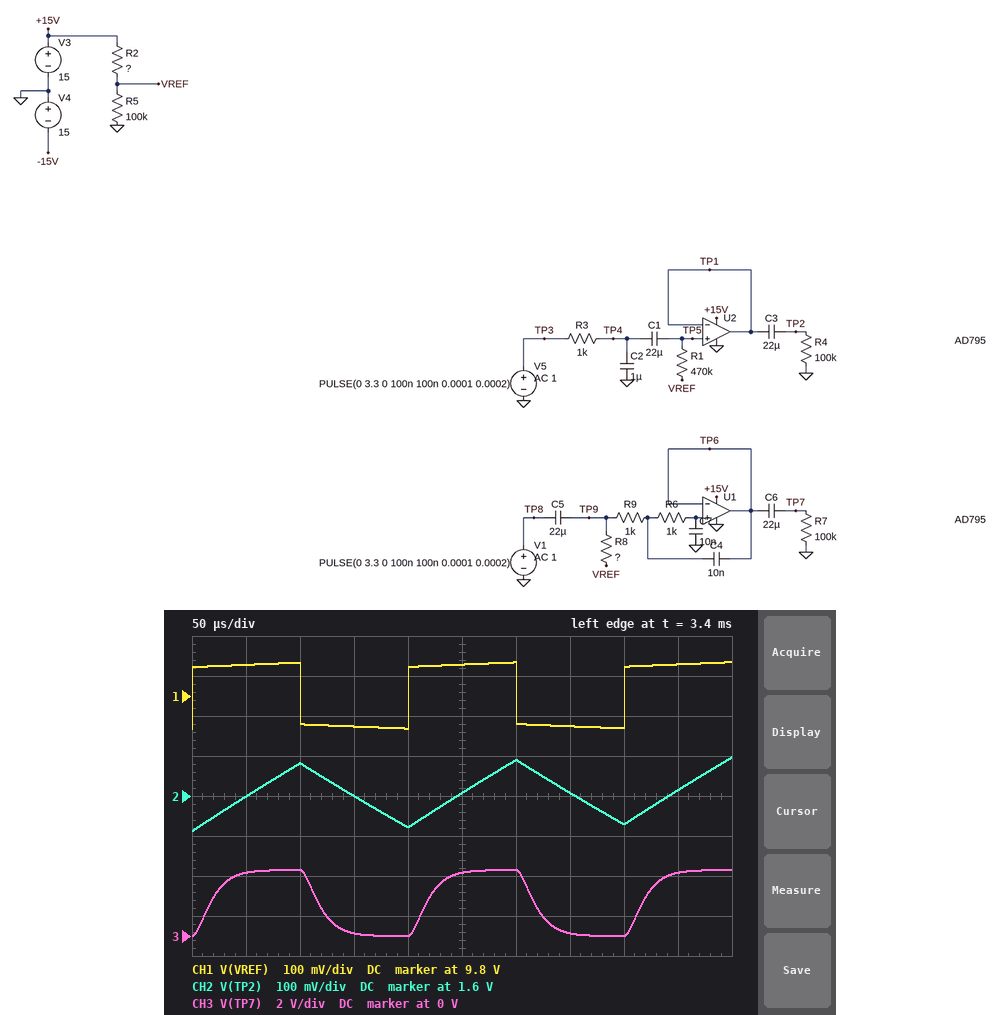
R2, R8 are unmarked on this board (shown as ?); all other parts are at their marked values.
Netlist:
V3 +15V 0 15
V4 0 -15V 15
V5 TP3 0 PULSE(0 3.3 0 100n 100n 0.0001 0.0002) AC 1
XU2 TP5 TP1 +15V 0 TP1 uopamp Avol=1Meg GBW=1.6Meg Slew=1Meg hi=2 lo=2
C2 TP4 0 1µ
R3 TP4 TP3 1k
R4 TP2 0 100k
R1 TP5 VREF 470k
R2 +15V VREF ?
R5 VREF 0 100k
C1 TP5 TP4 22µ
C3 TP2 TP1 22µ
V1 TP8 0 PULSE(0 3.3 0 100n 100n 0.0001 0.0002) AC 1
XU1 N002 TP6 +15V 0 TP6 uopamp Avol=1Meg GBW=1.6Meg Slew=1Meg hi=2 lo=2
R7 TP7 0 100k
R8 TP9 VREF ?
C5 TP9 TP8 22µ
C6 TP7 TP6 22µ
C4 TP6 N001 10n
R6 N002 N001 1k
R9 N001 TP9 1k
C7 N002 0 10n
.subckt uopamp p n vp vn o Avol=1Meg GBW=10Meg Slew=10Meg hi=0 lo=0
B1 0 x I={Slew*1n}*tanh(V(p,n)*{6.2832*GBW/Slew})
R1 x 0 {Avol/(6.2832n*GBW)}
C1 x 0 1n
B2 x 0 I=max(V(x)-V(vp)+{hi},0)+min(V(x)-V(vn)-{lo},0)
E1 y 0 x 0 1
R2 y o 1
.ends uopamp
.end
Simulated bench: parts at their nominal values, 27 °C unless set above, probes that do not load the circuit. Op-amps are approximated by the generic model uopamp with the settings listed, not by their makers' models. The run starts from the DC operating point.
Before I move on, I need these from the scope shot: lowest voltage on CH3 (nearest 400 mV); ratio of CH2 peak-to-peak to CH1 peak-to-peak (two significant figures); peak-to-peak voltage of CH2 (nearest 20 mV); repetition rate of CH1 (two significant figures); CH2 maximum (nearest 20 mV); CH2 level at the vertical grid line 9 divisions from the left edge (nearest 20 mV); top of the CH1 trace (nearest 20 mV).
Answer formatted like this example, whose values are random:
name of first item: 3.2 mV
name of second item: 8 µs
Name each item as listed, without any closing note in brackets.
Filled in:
lowest voltage on CH3: 0 V
ratio of CH2 peak-to-peak to CH1 peak-to-peak: 1.1
peak-to-peak voltage of CH2: 180 mV
repetition rate of CH1: 5.0 kHz
CH2 maximum: 1.70 V
CH2 level at the vertical grid line 9 divisions from the left edge: 1.62 V
top of the CH1 trace: 9.88 V
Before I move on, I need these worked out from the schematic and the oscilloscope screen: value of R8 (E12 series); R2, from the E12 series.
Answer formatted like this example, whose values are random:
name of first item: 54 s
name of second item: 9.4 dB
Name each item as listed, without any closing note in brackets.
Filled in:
value of R8: 680 kΩ
R2, from the E12 series: 56 kΩ
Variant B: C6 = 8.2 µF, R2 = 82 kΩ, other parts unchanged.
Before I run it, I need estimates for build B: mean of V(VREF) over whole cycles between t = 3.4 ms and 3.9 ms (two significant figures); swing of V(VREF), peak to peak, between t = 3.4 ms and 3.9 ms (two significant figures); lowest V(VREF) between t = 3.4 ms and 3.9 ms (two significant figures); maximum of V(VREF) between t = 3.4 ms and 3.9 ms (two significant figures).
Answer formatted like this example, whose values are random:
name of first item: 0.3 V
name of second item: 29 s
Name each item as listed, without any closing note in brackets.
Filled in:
mean of V(VREF) over whole cycles between t = 3.4 ms and 3.9 ms: 8.5 V
swing of V(VREF), peak to peak, between t = 3.4 ms and 3.9 ms: 200 mV
lowest V(VREF) between t = 3.4 ms and 3.9 ms: 8.4 V
maximum of V(VREF) between t = 3.4 ms and 3.9 ms: 8.6 V
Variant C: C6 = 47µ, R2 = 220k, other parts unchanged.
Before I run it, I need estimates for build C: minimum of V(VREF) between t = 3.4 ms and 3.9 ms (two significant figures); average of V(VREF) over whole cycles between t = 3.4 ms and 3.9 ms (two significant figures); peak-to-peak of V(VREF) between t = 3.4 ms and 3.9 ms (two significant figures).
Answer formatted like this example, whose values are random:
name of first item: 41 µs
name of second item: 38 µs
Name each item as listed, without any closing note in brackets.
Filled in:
minimum of V(VREF) between t = 3.4 ms and 3.9 ms: 4.9 V
average of V(VREF) over whole cycles between t = 3.4 ms and 3.9 ms: 5.0 V
peak-to-peak of V(VREF) between t = 3.4 ms and 3.9 ms: 290 mV
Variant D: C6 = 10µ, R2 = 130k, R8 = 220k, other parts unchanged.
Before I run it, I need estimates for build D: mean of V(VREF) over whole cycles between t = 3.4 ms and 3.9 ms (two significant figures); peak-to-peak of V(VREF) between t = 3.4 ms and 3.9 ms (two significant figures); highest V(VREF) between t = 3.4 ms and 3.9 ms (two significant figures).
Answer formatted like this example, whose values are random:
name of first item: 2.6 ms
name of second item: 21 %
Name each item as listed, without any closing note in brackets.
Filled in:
mean of V(VREF) over whole cycles between t = 3.4 ms and 3.9 ms: 7.0 V
peak-to-peak of V(VREF) between t = 3.4 ms and 3.9 ms: 630 mV
highest V(VREF) between t = 3.4 ms and 3.9 ms: 7.3 V
